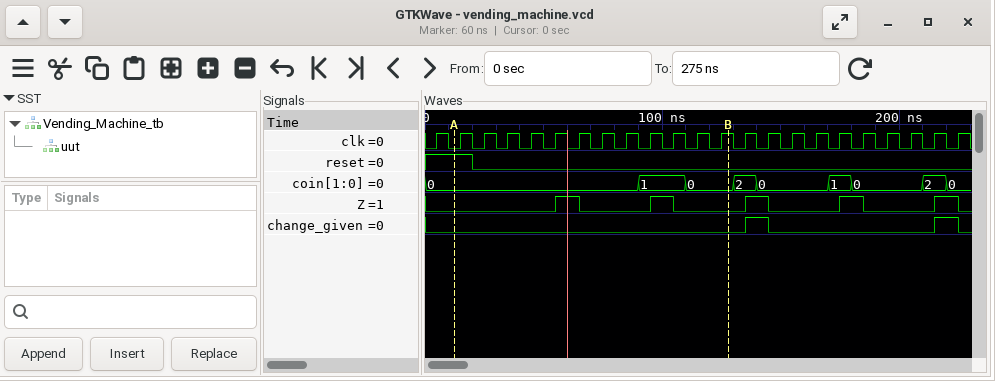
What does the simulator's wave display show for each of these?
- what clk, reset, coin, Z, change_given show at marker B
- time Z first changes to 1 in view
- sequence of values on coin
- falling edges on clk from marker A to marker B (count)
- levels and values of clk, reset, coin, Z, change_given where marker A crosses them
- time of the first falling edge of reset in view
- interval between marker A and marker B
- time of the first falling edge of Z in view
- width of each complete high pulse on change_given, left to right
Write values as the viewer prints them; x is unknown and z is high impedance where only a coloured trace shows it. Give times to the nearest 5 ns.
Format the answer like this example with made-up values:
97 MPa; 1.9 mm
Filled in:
clk=1, reset=0, coin=0, Z=0, change_given=0; 55 ns; 0, 1, 0, 2, 0, 1, 0, 2, 0; 11; clk=0, reset=1, coin=0, Z=0, change_given=0; 20 ns; 115 ns; 65 ns; 10 ns, 10 ns
